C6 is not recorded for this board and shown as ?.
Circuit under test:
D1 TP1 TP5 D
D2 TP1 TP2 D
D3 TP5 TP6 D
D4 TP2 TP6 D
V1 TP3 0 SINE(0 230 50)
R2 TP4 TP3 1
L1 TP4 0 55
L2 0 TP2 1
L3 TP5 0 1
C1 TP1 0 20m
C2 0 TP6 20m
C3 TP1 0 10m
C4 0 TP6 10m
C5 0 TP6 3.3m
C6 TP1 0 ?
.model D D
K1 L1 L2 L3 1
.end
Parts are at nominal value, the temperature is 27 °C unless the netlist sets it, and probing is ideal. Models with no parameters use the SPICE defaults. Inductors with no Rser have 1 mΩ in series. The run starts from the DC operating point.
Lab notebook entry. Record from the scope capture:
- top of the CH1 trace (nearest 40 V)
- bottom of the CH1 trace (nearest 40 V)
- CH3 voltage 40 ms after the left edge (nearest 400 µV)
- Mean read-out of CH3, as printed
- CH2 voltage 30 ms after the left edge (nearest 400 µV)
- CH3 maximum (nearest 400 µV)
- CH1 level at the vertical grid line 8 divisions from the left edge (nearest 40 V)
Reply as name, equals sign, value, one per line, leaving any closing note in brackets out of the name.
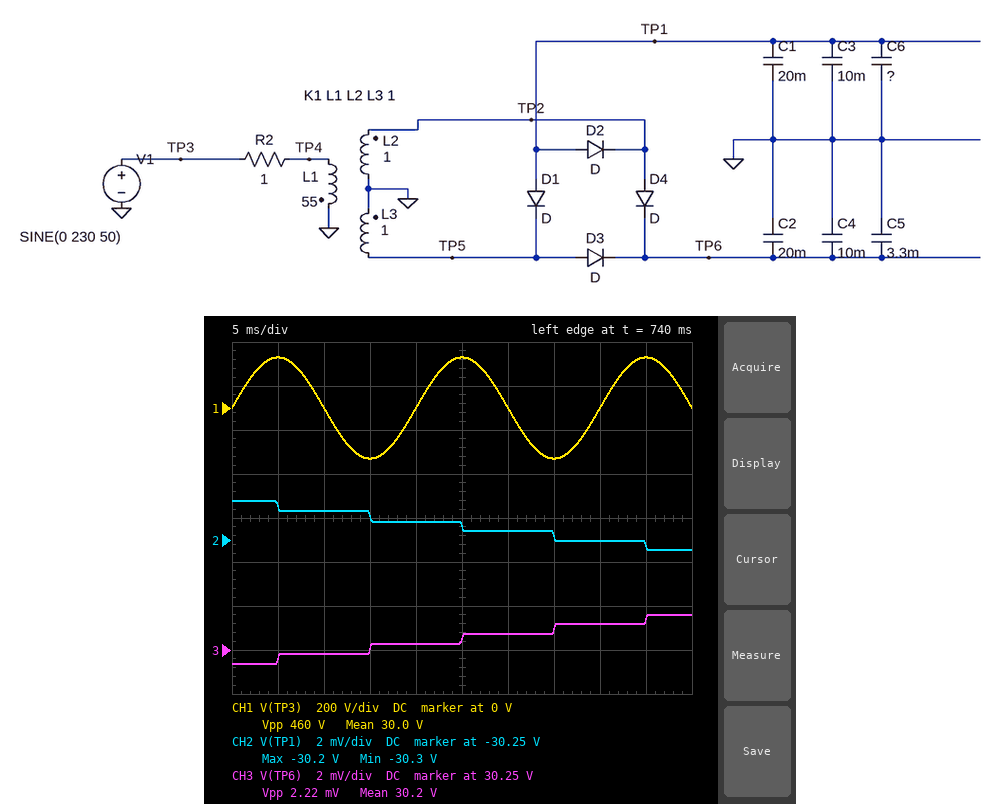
top of the CH1 trace = 240 V
bottom of the CH1 trace = -240 V
CH3 voltage 40 ms after the left edge = 30.2492 V
Mean read-out of CH3, as printed = 30.2 V
CH2 voltage 30 ms after the left edge = -30.2496 V
CH3 maximum = 30.2496 V
CH1 level at the vertical grid line 8 divisions from the left edge = 0 V
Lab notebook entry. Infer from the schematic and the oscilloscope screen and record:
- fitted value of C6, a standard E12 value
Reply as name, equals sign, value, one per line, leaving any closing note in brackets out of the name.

fitted value of C6, a standard E12 value = 2.2 mF
